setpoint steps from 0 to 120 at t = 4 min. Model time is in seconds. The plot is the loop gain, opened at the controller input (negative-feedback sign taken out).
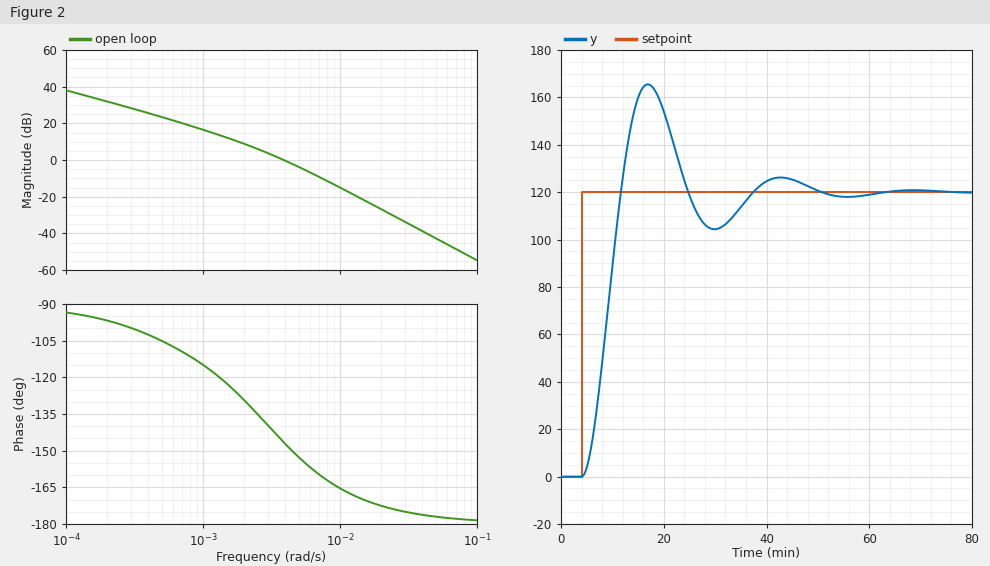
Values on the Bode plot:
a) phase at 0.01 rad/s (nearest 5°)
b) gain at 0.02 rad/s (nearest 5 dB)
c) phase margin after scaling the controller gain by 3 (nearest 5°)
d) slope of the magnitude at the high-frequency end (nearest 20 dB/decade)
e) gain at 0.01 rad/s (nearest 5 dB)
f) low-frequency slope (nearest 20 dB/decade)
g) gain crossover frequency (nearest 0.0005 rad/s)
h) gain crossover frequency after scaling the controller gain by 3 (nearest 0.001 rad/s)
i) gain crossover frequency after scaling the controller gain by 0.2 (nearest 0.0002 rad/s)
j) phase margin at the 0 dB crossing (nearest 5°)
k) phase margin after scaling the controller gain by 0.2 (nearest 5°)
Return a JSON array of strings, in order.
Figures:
["-165°", "-25 dB", "20°", "-40 dB/decade", "-15 dB", "-20 dB/decade", "0.0040 rad/s", "0.007 rad/s", "0.0012 rad/s", "35°", "60°"]
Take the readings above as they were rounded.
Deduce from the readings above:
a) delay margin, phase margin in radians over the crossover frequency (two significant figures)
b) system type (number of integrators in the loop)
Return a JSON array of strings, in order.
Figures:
["150 s", "1"]
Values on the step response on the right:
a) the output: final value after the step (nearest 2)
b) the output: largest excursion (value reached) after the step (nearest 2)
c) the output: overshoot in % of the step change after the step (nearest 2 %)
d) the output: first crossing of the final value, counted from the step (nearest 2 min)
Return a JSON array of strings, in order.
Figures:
["120", "166", "38 %", "8 min"]
